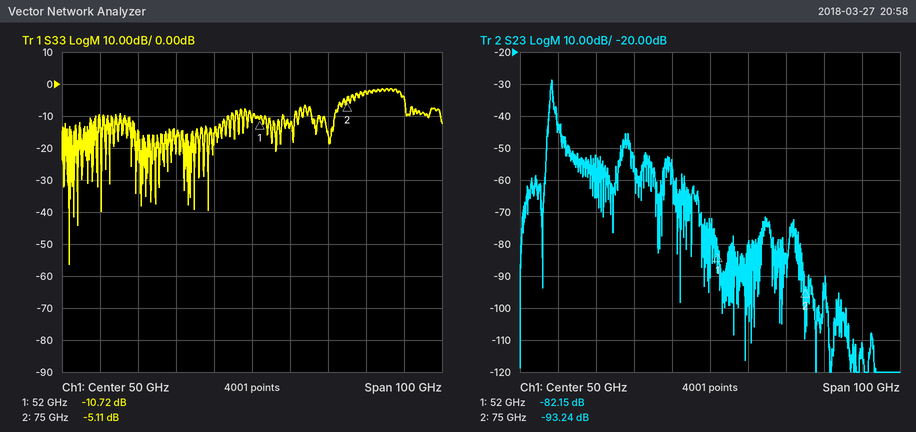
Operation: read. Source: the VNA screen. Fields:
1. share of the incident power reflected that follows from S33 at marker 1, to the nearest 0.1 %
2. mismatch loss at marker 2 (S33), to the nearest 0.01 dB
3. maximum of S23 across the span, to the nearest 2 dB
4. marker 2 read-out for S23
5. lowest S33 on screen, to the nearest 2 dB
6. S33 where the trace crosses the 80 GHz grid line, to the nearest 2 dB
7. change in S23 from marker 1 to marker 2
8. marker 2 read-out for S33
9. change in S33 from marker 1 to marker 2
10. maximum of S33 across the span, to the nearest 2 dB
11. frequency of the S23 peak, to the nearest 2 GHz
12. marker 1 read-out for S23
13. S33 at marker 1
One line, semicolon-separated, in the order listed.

8.5 %; 1.60 dB; -28 dB; -93.24 dB; -56 dB; -2 dB; -11.09 dB; -5.11 dB; 5.61 dB; -2 dB; 8 GHz; -82.15 dB; -10.72 dB
